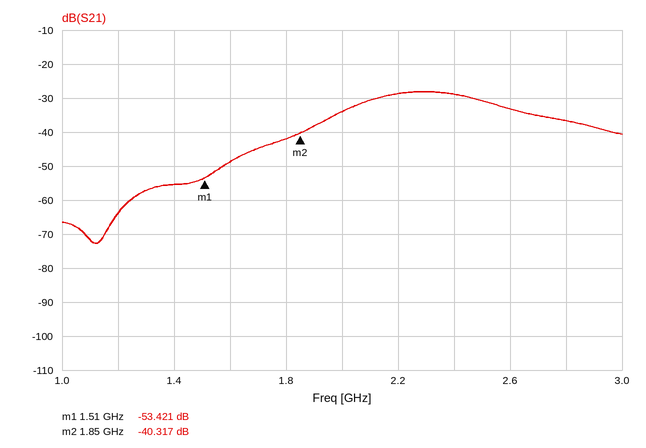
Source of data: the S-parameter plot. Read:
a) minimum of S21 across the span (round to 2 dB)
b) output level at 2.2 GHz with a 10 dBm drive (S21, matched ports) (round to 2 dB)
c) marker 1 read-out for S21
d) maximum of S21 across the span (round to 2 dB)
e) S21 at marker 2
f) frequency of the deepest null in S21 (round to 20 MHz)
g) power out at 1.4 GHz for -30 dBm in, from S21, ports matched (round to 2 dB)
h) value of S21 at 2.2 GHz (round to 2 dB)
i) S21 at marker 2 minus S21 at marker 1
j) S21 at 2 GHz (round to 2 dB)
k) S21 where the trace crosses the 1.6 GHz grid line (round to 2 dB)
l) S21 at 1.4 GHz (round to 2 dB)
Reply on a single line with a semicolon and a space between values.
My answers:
-72 dB; -18 dBm; -53.421 dB; -28 dB; -40.317 dB; 1.12 GHz; -86 dBm; -28 dB; 13.104 dB; -34 dB; -48 dB; -56 dB
